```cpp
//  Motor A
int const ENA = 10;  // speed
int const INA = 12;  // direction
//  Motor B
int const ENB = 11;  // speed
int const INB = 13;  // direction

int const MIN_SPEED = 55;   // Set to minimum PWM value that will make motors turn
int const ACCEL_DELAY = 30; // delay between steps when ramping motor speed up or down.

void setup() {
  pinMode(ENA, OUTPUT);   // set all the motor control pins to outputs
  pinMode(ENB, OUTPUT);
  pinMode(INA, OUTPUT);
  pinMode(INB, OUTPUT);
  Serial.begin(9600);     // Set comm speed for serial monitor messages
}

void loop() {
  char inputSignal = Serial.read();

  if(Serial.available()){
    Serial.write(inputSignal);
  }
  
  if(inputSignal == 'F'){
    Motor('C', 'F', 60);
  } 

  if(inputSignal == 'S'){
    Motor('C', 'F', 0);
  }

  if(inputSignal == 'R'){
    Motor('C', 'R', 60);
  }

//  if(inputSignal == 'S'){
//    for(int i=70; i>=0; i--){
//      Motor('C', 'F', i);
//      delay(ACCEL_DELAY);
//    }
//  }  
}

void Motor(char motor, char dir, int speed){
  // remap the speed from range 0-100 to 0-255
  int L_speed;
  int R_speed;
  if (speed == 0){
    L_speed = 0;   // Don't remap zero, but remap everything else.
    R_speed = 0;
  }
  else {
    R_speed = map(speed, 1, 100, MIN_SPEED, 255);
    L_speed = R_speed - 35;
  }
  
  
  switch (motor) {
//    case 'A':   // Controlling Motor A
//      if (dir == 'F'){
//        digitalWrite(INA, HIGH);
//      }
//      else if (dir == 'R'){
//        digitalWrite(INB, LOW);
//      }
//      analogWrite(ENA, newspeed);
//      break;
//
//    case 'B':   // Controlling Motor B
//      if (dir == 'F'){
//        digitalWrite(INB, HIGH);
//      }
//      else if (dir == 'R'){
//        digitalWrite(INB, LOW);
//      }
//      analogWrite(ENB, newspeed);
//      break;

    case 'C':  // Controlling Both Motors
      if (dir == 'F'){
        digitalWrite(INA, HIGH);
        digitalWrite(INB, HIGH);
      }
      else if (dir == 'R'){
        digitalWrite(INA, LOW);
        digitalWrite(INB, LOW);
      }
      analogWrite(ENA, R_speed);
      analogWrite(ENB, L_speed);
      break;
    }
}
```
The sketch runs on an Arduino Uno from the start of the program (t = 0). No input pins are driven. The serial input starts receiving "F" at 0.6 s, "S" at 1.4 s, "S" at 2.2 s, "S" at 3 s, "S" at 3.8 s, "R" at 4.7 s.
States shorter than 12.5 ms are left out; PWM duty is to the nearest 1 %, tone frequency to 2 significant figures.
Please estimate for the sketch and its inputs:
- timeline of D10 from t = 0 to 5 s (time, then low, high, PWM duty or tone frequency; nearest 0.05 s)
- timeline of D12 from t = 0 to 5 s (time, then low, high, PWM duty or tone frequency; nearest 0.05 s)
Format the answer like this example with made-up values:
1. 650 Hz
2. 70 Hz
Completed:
1. 0 s low; 0.6 s PWM 68 %; 1.4 s low; 4.7 s PWM 68 %
2. 0 s low; 0.6 s high; 4.7 s low
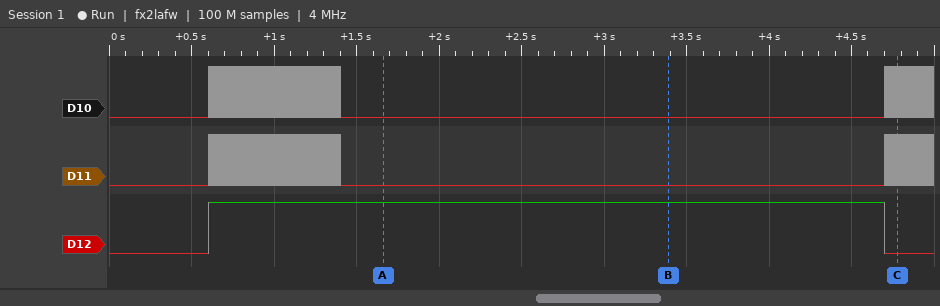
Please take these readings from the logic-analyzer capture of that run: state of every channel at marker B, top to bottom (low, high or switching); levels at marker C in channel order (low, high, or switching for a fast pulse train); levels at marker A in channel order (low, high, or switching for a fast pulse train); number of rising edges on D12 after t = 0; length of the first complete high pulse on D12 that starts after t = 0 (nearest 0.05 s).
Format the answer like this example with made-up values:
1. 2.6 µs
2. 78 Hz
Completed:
1. D10 low, D11 low, D12 high
2. D10 switching, D11 switching, D12 low
3. D10 low, D11 low, D12 high
4. 1
5. 4.10 s
